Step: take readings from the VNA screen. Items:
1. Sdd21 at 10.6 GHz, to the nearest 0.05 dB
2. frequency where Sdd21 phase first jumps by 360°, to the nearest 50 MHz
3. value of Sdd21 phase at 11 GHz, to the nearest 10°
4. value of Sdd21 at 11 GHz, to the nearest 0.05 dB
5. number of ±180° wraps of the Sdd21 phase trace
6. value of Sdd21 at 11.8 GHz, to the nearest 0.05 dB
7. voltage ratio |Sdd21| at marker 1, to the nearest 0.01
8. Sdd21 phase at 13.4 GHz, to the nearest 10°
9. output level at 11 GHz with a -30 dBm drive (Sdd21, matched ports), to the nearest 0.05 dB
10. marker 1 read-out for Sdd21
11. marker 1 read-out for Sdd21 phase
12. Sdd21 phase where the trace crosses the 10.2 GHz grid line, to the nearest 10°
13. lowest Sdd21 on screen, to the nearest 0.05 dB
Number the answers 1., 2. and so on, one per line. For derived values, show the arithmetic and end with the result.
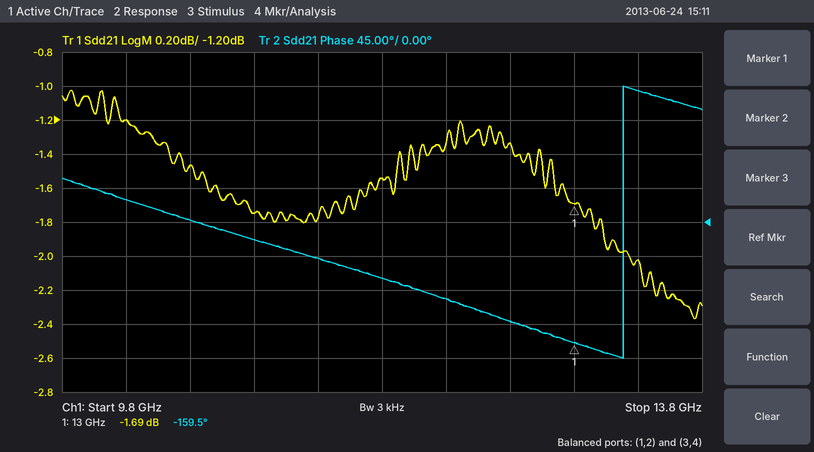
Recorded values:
1. -1.45 dB
2. 13.30 GHz
3. -20°
4. -1.75 dB
5. 1
6. -1.55 dB
7. 10^(-1.69/20) ≈ 0.82
8. 170°
9. -30 dBm + (-1.75 dB) = -31.75 dBm
10. -1.69 dB
11. -159.5°
12. 30°
13. -2.35 dB
